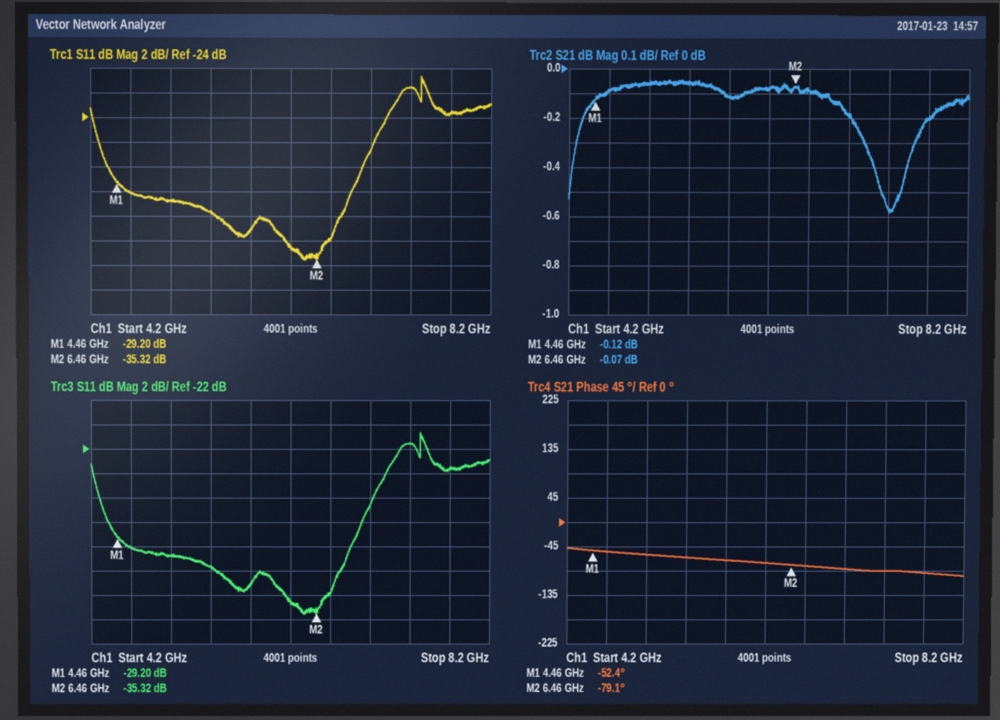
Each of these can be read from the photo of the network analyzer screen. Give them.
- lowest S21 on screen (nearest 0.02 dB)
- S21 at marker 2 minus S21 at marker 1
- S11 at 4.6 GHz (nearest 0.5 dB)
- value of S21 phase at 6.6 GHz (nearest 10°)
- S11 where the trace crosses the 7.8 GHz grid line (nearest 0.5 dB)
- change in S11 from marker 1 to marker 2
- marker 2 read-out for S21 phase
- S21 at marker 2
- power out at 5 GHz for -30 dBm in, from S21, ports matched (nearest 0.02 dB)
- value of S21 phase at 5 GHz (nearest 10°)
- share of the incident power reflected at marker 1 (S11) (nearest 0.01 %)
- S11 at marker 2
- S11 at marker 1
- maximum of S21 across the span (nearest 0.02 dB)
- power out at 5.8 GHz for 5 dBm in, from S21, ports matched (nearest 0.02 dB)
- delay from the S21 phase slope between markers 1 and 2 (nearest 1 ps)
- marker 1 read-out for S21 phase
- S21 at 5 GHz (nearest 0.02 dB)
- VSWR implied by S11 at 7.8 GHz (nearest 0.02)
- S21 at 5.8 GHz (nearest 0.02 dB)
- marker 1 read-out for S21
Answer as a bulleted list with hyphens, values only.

- -0.58 dB
- 0.05 dB
- -30.0 dB
- -80°
- -23.5 dB
- -6.12 dB
- -79.1°
- -0.07 dB
- -30.06 dBm
- -60°
- 0.12 %
- -35.32 dB
- -29.20 dB
- -0.04 dB
- 4.88 dBm
- 37 ps
- -52.4°
- -0.06 dB
- 1.14
- -0.12 dB
- -0.12 dB
